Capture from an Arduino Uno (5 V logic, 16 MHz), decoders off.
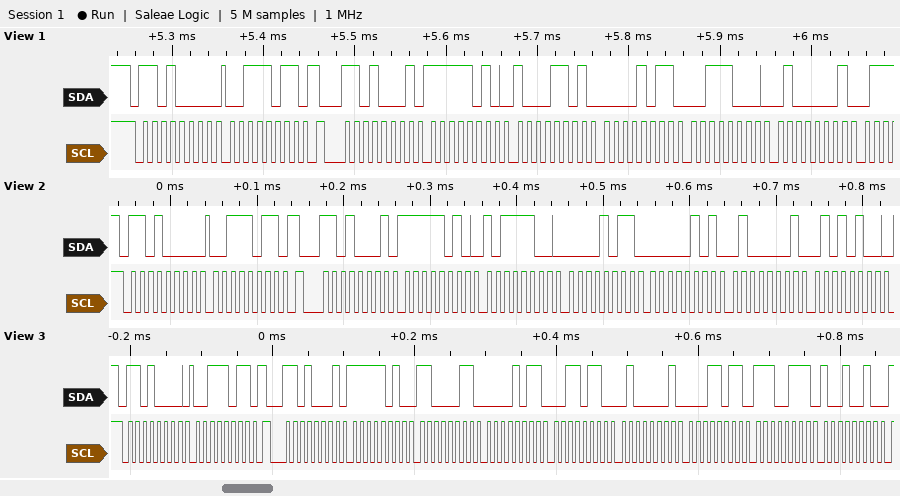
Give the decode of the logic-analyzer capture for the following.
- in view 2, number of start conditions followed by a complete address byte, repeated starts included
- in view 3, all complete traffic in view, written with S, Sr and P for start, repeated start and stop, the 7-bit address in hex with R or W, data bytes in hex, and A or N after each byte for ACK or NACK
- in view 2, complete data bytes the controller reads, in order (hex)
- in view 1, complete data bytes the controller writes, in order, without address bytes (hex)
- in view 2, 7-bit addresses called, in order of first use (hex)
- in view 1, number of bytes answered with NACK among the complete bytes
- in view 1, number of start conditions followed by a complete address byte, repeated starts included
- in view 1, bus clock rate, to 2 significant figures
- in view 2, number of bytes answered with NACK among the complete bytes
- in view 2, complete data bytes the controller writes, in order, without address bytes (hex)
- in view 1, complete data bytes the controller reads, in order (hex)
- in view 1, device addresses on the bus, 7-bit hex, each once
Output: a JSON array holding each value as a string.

["2", "S 68W A 3B A Sr 68R A FA A C3 A 0B A 36 A 41 A 1B A E7 A 92 A", "FA BC 0B 05 41 54", "3B", "0x68", "0", "2", "100 kHz", "0", "3B", "FA 8D 0B 38 41", "0x68"]
